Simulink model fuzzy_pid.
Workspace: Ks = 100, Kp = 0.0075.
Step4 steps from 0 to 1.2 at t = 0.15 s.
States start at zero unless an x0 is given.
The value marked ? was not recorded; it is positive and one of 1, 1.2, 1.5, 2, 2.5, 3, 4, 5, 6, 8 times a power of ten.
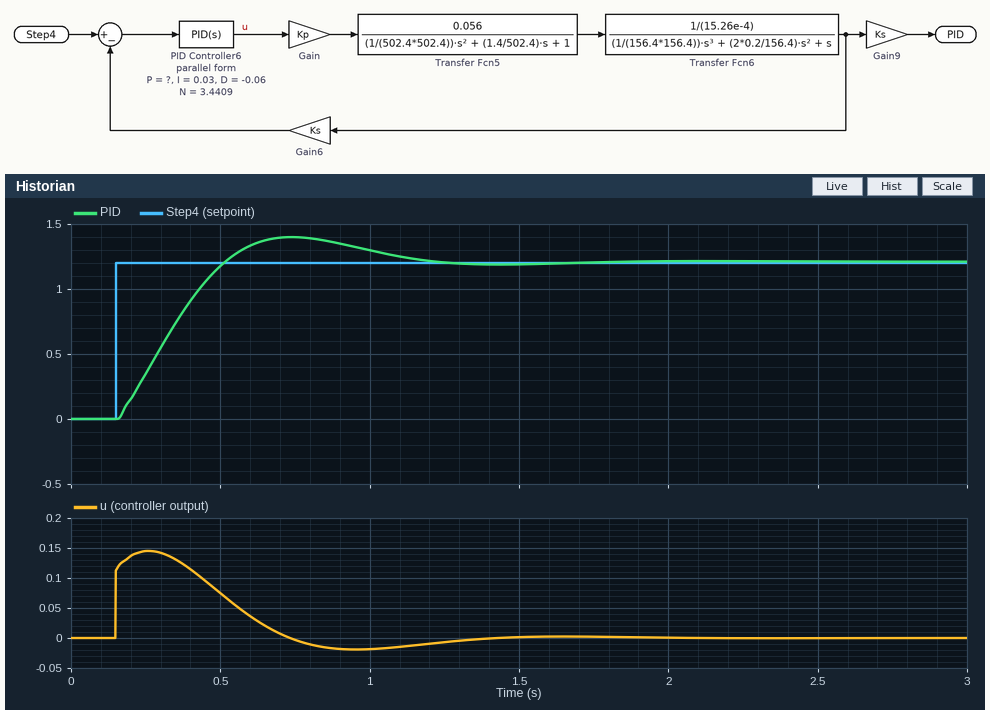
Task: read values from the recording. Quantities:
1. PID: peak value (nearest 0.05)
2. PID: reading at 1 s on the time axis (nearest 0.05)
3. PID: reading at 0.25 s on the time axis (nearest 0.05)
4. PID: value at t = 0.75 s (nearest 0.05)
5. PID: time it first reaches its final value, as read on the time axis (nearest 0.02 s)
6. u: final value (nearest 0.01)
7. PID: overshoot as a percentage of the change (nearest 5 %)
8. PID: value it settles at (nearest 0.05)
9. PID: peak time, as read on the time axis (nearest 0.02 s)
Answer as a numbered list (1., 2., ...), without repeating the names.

1. 1.40
2. 1.30
3. 0.35
4. 1.40
5. 0.52 s
6. 0.00
7. 15 %
8. 1.20
9. 0.74 s
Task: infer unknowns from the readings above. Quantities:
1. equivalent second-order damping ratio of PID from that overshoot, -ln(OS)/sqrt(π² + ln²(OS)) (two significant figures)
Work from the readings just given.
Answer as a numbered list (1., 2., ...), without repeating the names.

1. 0.52
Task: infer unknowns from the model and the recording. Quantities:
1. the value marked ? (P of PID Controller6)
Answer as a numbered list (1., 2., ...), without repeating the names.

1. 0.3
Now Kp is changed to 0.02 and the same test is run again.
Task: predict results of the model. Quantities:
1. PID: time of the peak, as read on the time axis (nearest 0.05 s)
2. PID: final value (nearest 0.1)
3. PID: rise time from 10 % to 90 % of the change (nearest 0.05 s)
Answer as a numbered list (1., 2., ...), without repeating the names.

1. 0.45 s
2. 1.2
3. 0.15 s
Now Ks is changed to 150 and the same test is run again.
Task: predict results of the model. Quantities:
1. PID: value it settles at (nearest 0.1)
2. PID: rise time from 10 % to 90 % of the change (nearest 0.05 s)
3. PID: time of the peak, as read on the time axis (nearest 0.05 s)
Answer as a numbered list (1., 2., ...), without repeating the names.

1. 1.2
2. 0.20 s
3. 0.60 s
